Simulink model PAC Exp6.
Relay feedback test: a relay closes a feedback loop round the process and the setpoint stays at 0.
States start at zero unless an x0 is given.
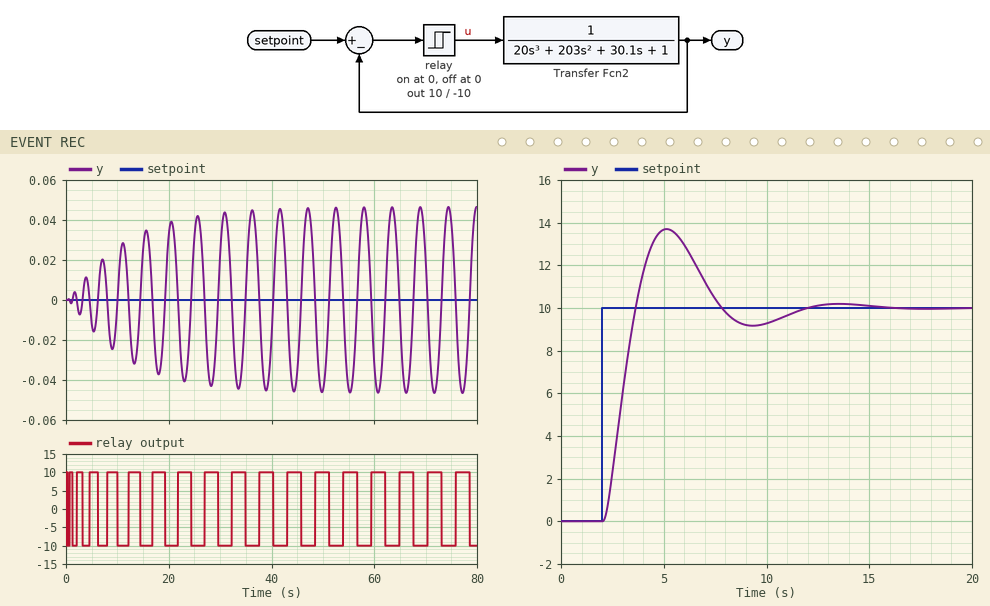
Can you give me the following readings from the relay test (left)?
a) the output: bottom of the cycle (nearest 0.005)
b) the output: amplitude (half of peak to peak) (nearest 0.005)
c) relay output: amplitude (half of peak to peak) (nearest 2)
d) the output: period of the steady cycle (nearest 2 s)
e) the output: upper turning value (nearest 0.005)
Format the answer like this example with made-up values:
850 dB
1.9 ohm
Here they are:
-0.045
0.045
10
6 s
0.045
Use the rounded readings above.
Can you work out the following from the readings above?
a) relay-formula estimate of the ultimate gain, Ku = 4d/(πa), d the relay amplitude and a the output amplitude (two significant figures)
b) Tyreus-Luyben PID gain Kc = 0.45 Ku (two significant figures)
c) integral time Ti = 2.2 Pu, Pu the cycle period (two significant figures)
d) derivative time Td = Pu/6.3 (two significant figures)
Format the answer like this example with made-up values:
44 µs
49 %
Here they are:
280
130
13 s
0.95 s
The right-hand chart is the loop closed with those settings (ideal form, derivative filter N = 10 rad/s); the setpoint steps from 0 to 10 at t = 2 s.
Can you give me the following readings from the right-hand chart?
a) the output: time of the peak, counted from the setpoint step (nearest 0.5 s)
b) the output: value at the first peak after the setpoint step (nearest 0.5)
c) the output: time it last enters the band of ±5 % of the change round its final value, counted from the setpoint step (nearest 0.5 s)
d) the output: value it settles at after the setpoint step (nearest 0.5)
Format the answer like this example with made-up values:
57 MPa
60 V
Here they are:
3.0 s
13.5
8.5 s
10.0
